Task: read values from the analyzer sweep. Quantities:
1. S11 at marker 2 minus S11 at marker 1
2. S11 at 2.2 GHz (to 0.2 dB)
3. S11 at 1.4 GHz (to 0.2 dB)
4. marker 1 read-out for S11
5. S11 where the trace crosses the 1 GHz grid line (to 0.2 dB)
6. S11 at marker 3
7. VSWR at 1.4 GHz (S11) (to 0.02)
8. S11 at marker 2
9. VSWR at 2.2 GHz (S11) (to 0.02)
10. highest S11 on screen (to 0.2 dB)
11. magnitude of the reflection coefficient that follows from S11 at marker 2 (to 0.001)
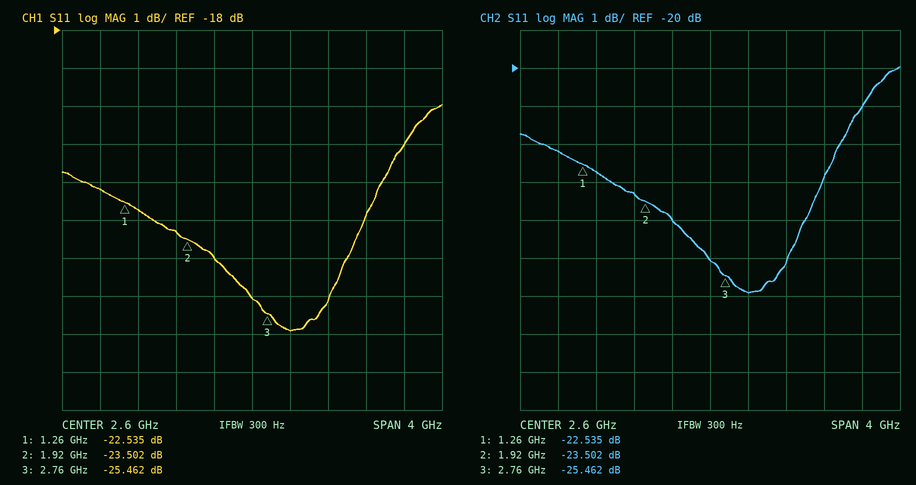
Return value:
-0.967 dB
-24.0 dB
-22.8 dB
-22.535 dB
-22.2 dB
-25.462 dB
1.16
-23.502 dB
1.14
-20.0 dB
0.067
